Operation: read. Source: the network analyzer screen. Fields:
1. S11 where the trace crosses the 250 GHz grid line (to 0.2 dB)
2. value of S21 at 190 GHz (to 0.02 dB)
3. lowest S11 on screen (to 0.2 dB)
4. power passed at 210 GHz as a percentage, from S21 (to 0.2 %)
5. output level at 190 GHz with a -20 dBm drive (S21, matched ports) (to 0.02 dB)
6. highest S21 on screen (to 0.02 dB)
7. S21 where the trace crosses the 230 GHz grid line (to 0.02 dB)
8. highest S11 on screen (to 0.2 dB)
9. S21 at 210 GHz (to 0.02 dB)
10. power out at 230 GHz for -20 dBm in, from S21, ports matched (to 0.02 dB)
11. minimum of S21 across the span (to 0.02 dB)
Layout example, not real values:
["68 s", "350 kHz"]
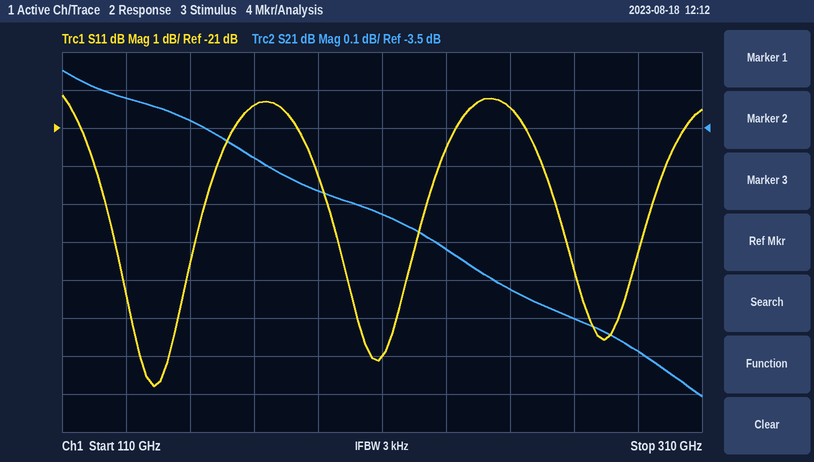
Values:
["-20.4 dB", "-3.66 dB", "-27.8 dB", "42.4 %", "-23.66 dBm", "-3.34 dB", "-3.82 dB", "-20.2 dB", "-3.72 dB", "-23.82 dBm", "-4.20 dB"]
